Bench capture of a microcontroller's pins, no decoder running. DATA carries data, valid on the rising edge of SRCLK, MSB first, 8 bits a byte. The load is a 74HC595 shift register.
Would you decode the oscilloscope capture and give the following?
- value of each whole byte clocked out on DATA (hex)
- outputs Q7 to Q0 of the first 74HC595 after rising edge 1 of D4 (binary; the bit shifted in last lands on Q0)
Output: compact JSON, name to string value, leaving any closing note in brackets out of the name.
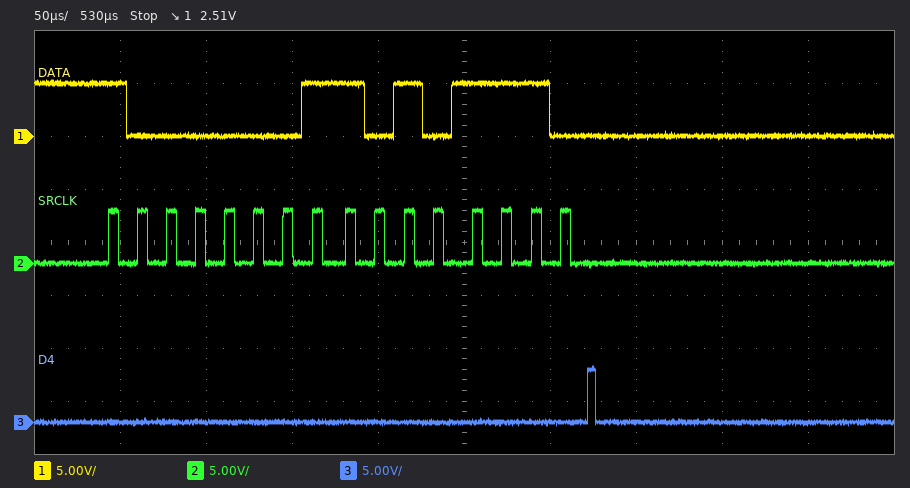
{"value of each whole byte clocked out on DATA": "0x81 0xAE", "outputs Q7 to Q0 of the first 74HC595 after rising edge 1 of D4": "10101110"}
